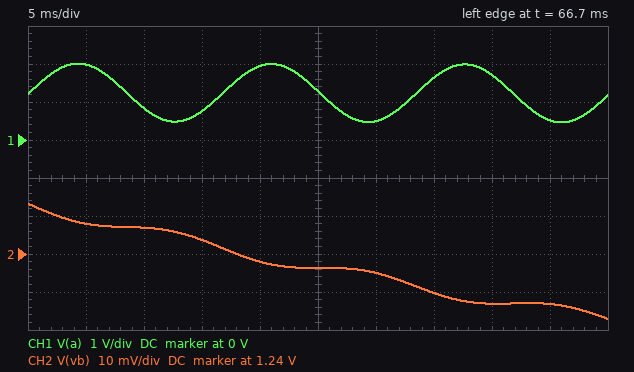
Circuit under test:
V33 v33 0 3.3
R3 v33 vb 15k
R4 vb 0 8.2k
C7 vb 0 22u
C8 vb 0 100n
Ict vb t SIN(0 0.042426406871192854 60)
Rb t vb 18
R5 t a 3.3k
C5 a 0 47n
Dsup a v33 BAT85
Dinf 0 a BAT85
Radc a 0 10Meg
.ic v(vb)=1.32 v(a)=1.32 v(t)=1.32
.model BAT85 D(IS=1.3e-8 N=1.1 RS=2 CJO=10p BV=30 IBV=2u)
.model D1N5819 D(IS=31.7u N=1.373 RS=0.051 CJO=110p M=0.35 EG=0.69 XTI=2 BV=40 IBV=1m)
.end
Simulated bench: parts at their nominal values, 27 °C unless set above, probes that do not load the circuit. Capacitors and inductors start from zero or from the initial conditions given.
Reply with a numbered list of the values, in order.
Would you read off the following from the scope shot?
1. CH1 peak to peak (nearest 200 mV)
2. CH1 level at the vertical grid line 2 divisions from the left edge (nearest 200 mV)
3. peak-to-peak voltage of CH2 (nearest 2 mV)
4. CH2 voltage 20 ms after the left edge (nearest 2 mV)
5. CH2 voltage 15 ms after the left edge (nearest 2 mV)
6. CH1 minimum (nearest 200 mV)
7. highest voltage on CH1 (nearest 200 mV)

1. 1.6 V
2. 800 mV
3. 30 mV
4. 1.238 V
5. 1.244 V
6. 400 mV
7. 2.0 V
